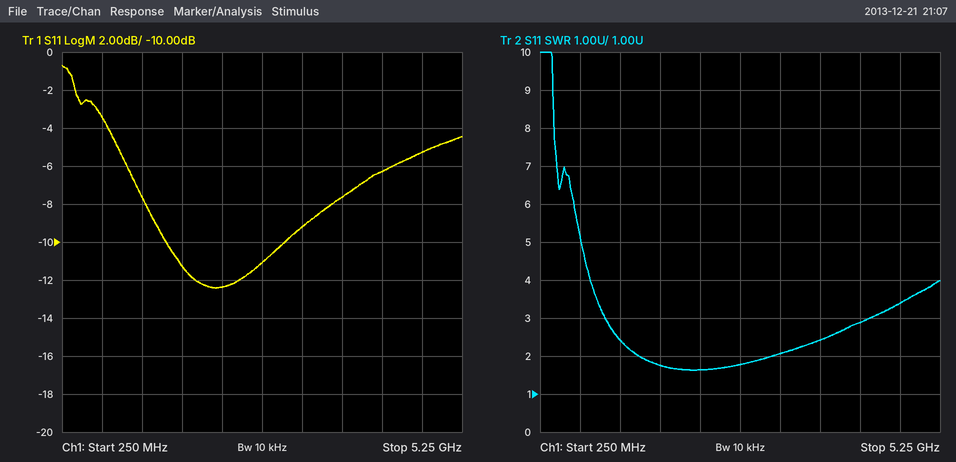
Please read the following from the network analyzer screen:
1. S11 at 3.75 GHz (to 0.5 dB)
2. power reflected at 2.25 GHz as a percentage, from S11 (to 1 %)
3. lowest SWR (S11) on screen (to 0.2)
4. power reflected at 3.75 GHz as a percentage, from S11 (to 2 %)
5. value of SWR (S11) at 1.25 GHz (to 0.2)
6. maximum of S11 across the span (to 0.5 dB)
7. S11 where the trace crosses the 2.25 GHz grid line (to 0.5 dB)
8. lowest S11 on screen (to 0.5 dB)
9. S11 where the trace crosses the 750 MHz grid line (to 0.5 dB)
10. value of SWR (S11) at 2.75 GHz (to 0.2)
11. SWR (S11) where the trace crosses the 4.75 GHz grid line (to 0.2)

-7.5 dB
6 %
1.6
18 %
2.4
-0.5 dB
-12.5 dB
-12.5 dB
-3.5 dB
1.8
3.4
